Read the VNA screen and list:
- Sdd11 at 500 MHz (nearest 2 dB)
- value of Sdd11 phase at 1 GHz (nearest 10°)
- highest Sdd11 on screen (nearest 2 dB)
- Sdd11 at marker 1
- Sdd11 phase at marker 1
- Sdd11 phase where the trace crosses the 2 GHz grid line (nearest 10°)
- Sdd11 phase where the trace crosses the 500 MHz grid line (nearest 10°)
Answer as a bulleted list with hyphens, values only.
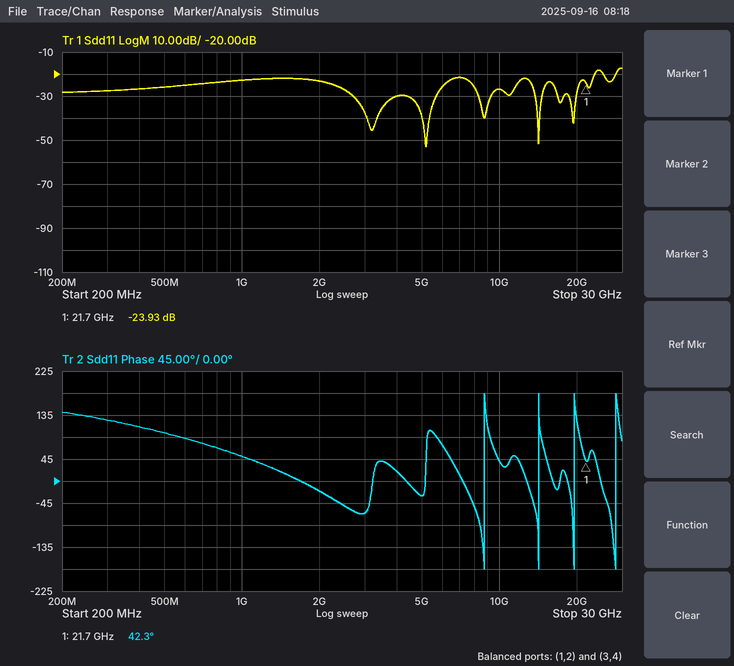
- -26 dB
- 50°
- -18 dB
- -23.93 dB
- 42.3°
- -20°
- 100°
